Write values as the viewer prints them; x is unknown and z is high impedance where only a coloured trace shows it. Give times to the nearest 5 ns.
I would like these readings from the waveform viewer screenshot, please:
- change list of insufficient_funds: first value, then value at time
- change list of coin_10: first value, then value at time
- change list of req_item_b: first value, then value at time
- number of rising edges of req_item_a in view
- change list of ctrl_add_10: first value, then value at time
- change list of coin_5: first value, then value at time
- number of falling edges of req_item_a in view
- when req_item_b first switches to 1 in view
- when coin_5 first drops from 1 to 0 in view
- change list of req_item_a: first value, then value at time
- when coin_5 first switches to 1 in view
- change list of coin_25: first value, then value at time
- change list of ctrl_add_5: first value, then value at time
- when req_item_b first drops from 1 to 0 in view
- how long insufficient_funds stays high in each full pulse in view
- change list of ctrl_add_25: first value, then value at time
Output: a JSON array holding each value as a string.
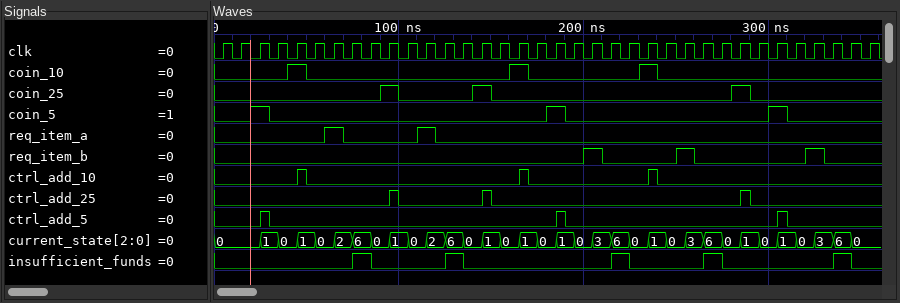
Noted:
["0, 1 at 75 ns, 0 at 85 ns, 1 at 125 ns, 0 at 135 ns, 1 at 215 ns, 0 at 225 ns, 1 at 265 ns, 0 at 275 ns, 1 at 335 ns, 0 at 345 ns", "0, 1 at 40 ns, 0 at 50 ns, 1 at 160 ns, 0 at 170 ns, 1 at 230 ns, 0 at 240 ns", "0, 1 at 200 ns, 0 at 210 ns, 1 at 250 ns, 0 at 260 ns, 1 at 320 ns, 0 at 330 ns", "2", "0, 1 at 45 ns, 0 at 50 ns, 1 at 165 ns, 0 at 170 ns, 1 at 235 ns, 0 at 240 ns", "0, 1 at 20 ns, 0 at 30 ns, 1 at 180 ns, 0 at 190 ns, 1 at 300 ns, 0 at 310 ns", "2", "200 ns", "30 ns", "0, 1 at 60 ns, 0 at 70 ns, 1 at 110 ns, 0 at 120 ns", "20 ns", "0, 1 at 90 ns, 0 at 100 ns, 1 at 140 ns, 0 at 150 ns, 1 at 280 ns, 0 at 290 ns", "0, 1 at 25 ns, 0 at 30 ns, 1 at 185 ns, 0 at 190 ns, 1 at 305 ns, 0 at 310 ns", "210 ns", "10 ns, 10 ns, 10 ns, 10 ns, 10 ns", "0, 1 at 95 ns, 0 at 100 ns, 1 at 145 ns, 0 at 150 ns, 1 at 285 ns, 0 at 290 ns"]
